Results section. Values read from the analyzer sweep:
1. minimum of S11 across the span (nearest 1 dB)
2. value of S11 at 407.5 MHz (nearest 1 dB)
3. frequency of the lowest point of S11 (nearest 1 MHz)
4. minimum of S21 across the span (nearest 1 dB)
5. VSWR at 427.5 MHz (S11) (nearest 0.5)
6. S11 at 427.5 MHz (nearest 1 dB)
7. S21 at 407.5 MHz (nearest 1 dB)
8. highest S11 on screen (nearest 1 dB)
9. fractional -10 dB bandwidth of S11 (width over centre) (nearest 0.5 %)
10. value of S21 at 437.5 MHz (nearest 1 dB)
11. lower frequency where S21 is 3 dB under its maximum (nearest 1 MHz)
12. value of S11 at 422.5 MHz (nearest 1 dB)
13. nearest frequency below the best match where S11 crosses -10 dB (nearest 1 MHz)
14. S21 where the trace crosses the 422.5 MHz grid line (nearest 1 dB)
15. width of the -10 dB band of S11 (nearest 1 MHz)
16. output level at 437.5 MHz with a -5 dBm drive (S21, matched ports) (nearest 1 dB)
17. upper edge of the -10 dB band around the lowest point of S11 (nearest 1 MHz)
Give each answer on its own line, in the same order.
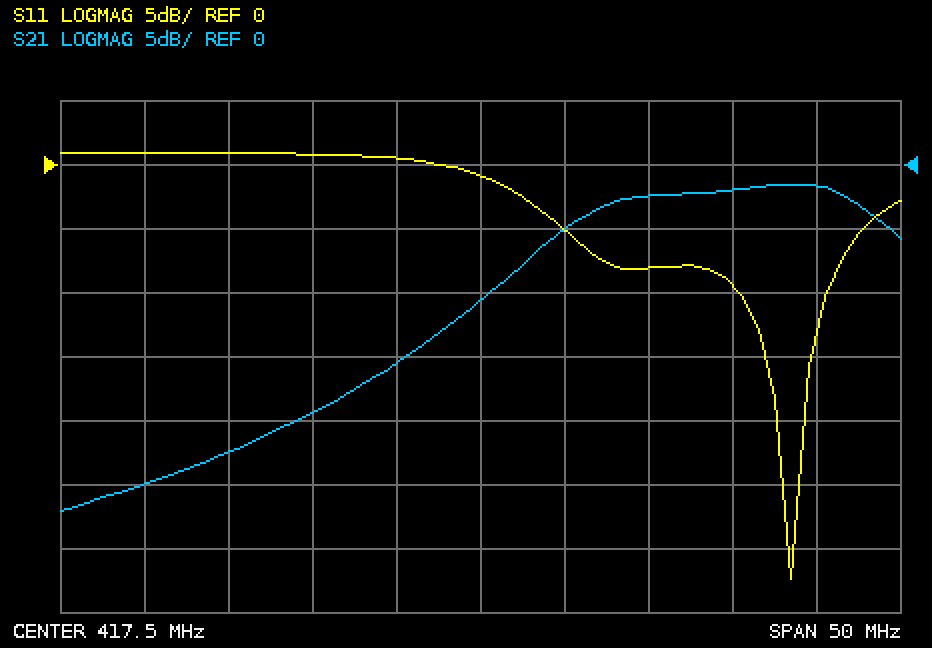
-32 dB
1 dB
436 MHz
-27 dB
2.5
-8 dB
-19 dB
1 dB
1.0 %
-2 dB
423 MHz
-5 dB
433 MHz
-5 dB
5 MHz
-7 dBm
438 MHz
